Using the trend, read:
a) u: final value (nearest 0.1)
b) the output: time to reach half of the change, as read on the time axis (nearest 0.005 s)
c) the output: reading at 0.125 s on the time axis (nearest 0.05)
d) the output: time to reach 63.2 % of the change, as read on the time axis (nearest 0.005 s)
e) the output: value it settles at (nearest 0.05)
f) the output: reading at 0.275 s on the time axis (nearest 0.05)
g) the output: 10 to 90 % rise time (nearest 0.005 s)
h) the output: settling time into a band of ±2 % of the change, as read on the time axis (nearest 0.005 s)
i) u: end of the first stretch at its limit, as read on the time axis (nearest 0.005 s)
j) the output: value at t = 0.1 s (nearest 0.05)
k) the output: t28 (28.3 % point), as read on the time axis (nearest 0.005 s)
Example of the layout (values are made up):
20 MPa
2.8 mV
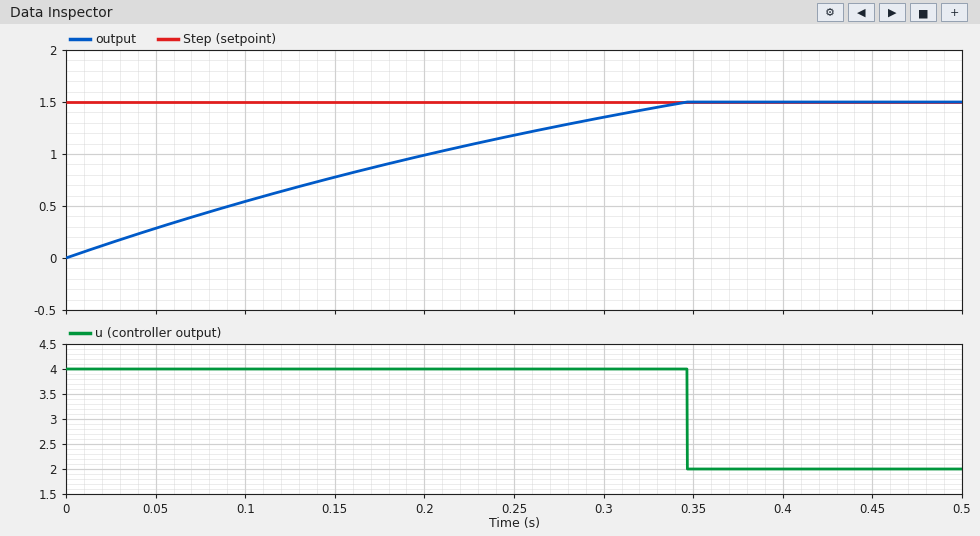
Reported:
2.0
0.145 s
0.65
0.190 s
1.50
1.25
0.275 s
0.335 s
0.345 s
0.55
0.075 s
